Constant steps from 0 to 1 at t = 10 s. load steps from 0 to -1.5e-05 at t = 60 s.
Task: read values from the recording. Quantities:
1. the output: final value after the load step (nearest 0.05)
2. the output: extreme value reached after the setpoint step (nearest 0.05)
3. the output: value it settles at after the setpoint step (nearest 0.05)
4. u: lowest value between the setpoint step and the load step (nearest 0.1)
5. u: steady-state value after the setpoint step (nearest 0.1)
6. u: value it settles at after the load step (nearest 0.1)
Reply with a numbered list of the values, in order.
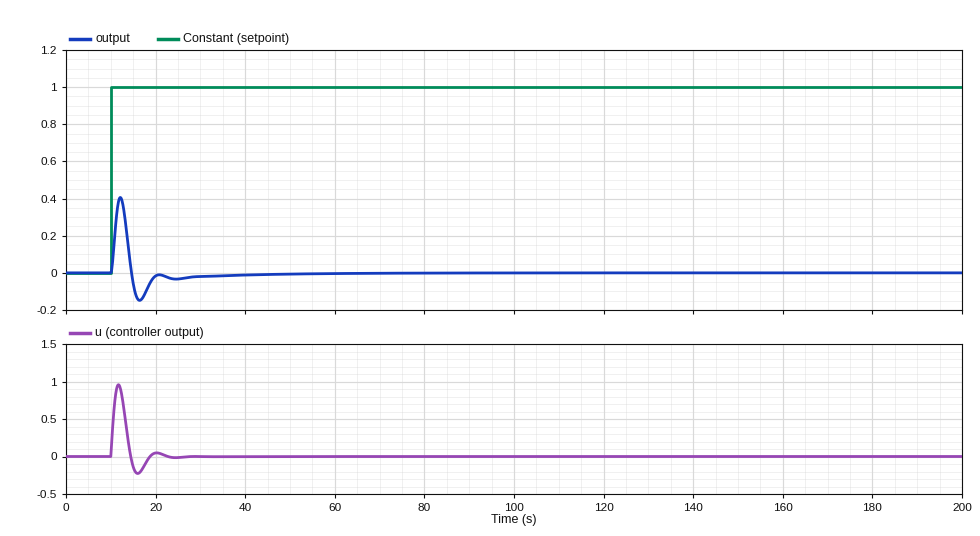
1. 0.00
2. 0.40
3. 0.00
4. -0.2
5. 0.0
6. 0.0
